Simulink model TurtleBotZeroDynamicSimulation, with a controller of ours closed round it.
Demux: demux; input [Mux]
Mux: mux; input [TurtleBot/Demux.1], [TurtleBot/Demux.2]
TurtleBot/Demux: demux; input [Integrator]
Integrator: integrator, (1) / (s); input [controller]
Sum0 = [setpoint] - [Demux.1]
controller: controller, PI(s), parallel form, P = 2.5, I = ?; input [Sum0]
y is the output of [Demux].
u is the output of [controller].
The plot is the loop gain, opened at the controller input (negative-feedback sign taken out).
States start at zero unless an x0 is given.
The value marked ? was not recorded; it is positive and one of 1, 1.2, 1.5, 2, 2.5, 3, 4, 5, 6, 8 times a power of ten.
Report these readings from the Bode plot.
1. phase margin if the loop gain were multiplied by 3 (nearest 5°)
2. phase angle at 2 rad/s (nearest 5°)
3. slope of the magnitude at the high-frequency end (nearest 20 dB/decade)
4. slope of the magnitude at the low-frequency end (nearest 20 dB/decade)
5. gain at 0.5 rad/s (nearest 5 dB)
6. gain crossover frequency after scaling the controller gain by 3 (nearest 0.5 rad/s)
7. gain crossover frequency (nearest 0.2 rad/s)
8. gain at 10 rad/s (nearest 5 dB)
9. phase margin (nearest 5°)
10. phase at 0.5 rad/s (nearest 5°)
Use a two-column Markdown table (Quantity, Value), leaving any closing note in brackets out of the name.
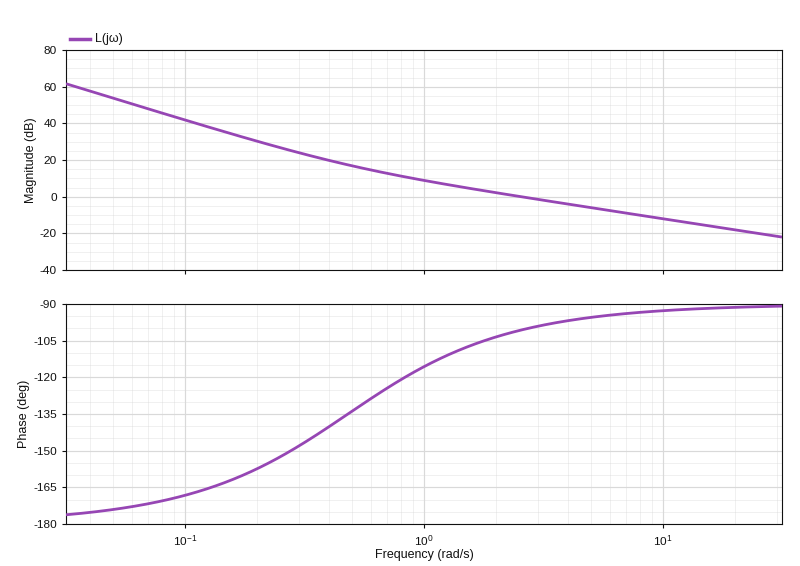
| Quantity | Value |
|---|---|
| phase margin if the loop gain were multiplied by 3 | 85° |
| phase angle at 2 rad/s | -105° |
| slope of the magnitude at the high-frequency end | -20 dB/decade |
| slope of the magnitude at the low-frequency end | -40 dB/decade |
| gain at 0.5 rad/s | 15 dB |
| gain crossover frequency after scaling the controller gain by 3 | 7.5 rad/s |
| gain crossover frequency | 2.6 rad/s |
| gain at 10 rad/s | -10 dB |
| phase margin | 80° |
| phase at 0.5 rad/s | -135° |
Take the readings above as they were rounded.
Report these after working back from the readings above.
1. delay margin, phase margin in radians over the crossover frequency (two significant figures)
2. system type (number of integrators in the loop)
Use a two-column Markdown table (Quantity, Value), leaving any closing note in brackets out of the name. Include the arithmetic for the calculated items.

| Quantity | Value |
|---|---|
| delay margin, phase margin in radians over the crossover frequency | 80 × π / 180 / 2.6 = 0.54 s |
| system type | 2 |
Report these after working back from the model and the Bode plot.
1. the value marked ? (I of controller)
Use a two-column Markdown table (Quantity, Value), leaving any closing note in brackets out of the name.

| Quantity | Value |
|---|---|
| the value marked ? | 1.2 |
